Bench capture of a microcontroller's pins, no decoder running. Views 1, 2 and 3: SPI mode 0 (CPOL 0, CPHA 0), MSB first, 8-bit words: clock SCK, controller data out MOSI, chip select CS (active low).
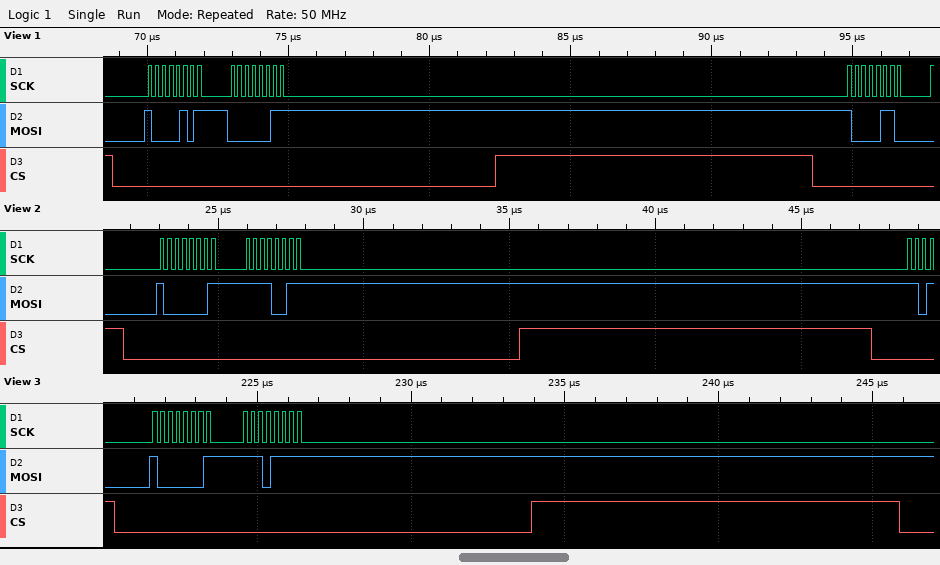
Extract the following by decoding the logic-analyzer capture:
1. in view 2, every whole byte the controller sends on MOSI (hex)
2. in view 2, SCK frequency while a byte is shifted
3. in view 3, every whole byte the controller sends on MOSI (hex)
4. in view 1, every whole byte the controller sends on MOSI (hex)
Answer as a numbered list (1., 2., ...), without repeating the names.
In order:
1. 81 F3
2. 4 MHz
3. 0x81 0xEF
4. 85 03 86
